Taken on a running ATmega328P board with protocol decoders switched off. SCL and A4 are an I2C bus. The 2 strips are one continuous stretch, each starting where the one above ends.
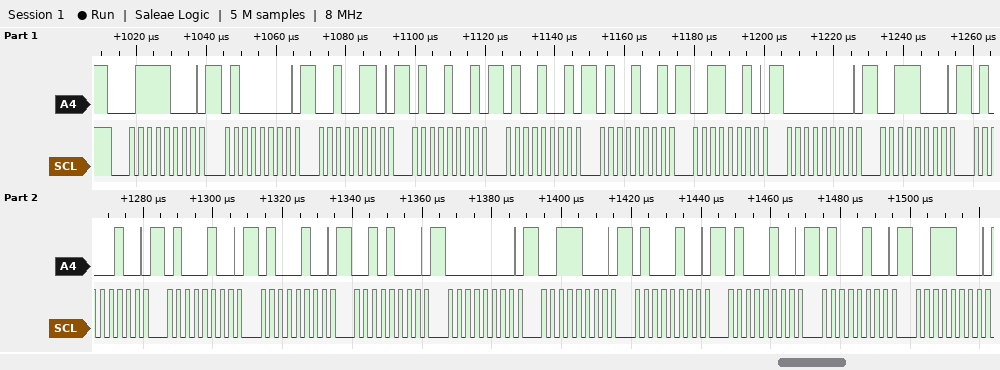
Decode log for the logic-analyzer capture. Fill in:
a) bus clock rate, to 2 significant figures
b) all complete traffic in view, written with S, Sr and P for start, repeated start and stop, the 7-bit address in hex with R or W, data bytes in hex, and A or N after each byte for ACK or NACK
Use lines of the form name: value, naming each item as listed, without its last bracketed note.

bus clock rate, to 2 significant figures: 400 kHz
all complete traffic in view, written with S, Sr and P for start, repeated start and stop, the 7-bit address in hex with R or W, data bytes in hex, and A or N after each byte for ACK or NACK: S 3CW A 40 A 26 A 49 A 49 A 49 A 32 A 00 A 38 A 44 A 44 A 44 A 28 A 00 A 38 A 44 A 44 A 44 A 38 A
